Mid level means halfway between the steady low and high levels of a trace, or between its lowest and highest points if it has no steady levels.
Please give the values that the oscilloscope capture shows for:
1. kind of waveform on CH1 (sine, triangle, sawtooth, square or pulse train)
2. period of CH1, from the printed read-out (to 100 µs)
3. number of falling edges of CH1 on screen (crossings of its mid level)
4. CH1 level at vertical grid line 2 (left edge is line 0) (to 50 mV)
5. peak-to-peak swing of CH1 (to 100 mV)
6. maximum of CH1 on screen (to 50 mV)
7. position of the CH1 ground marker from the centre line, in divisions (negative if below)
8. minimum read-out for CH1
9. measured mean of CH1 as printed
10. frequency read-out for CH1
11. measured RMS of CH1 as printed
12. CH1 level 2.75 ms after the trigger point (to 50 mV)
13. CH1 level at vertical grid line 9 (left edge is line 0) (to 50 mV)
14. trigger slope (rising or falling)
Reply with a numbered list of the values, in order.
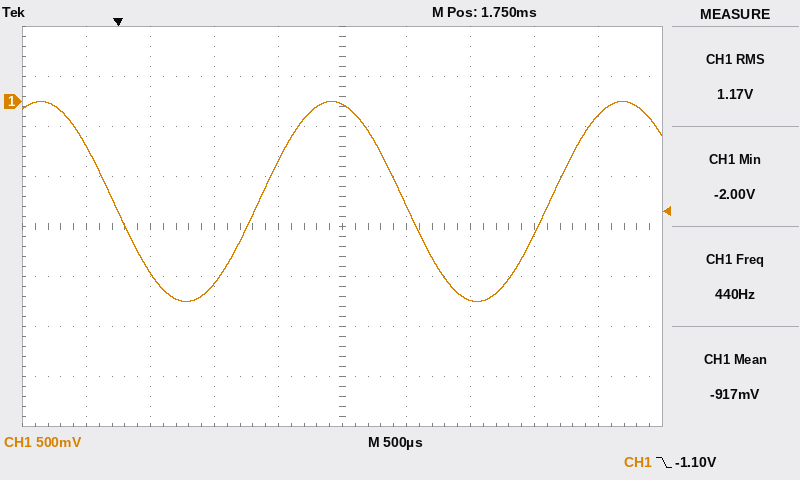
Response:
1. sine
2. 2.3 ms
3. 2
4. -1.70 V
5. 2.00 V
6. 0 mV
7. +2.5 div
8. -2.00 V
9. -917 mV
10. 440 Hz
11. 1.17 V
12. -2.00 V
13. -150 mV
14. falling
